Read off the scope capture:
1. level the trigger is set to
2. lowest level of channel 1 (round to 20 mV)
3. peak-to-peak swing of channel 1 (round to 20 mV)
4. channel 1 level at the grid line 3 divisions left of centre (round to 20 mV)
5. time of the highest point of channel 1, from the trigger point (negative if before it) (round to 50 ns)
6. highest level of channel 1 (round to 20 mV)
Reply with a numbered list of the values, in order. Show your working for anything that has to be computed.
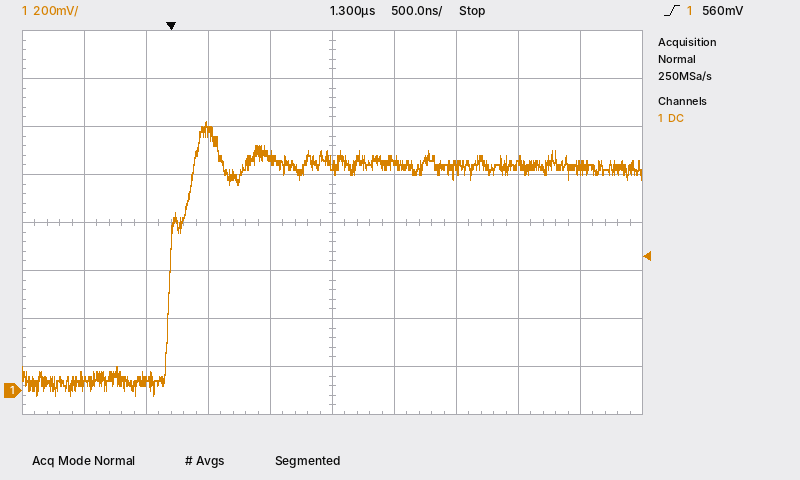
1. 560 mV
2. -20 mV
3. 1.12 V − (-20 mV) = 1.14 V
4. 40 mV
5. +300 ns
6. 1.12 V
